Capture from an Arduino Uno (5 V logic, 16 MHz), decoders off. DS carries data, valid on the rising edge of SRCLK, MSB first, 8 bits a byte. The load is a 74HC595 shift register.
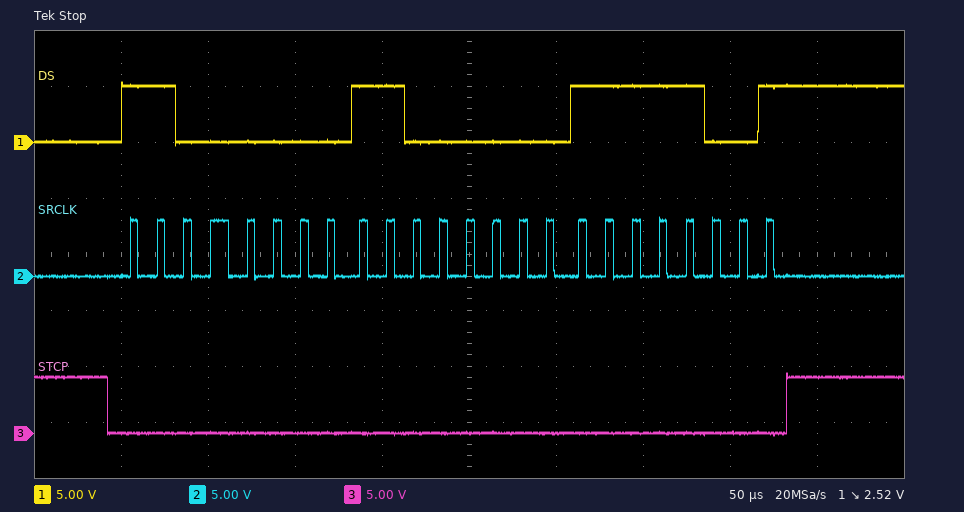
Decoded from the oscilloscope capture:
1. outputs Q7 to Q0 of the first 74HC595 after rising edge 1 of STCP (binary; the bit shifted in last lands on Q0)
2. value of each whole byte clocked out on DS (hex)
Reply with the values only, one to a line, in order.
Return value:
11111001
0xC0 0xC0 0xF9
